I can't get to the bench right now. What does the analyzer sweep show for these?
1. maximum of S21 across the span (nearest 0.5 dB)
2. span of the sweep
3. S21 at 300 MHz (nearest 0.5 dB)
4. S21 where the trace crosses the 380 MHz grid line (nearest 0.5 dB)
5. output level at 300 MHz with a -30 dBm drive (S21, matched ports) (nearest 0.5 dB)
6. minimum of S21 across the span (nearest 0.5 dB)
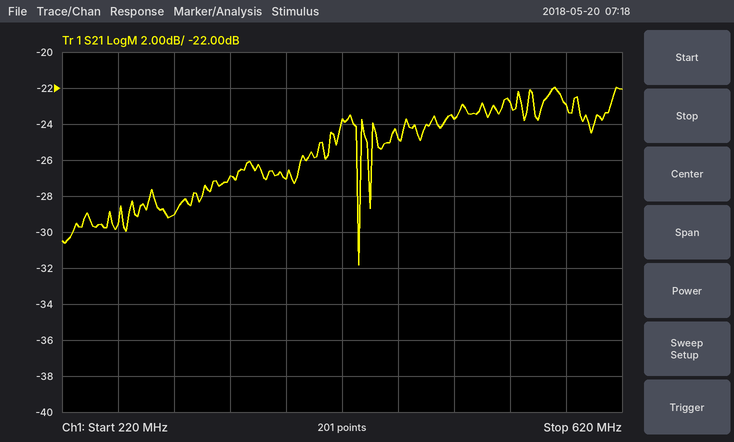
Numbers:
-22.0 dB
400 MHz
-29.0 dB
-27.0 dB
-59.0 dBm
-32.0 dB
